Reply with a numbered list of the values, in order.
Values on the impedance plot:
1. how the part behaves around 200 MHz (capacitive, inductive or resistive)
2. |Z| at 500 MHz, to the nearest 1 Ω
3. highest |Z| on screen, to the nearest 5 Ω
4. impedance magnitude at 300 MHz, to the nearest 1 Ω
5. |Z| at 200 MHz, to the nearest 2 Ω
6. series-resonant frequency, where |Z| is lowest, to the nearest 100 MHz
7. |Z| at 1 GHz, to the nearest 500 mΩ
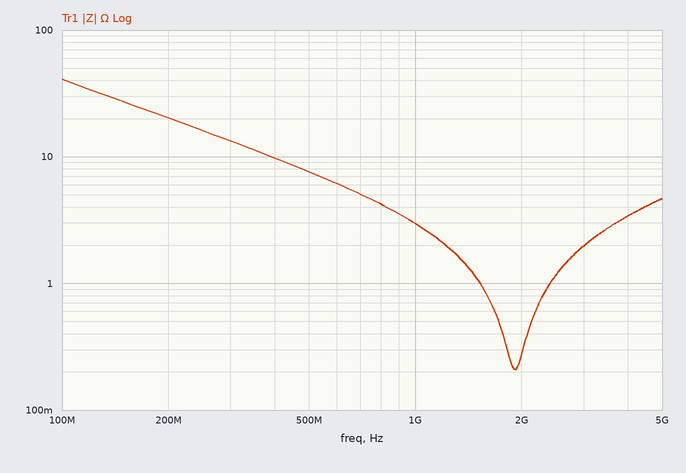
1. capacitive
2. 8 Ω
3. 40 Ω
4. 13 Ω
5. 20 Ω
6. 1.9 GHz
7. 3.0 Ω
